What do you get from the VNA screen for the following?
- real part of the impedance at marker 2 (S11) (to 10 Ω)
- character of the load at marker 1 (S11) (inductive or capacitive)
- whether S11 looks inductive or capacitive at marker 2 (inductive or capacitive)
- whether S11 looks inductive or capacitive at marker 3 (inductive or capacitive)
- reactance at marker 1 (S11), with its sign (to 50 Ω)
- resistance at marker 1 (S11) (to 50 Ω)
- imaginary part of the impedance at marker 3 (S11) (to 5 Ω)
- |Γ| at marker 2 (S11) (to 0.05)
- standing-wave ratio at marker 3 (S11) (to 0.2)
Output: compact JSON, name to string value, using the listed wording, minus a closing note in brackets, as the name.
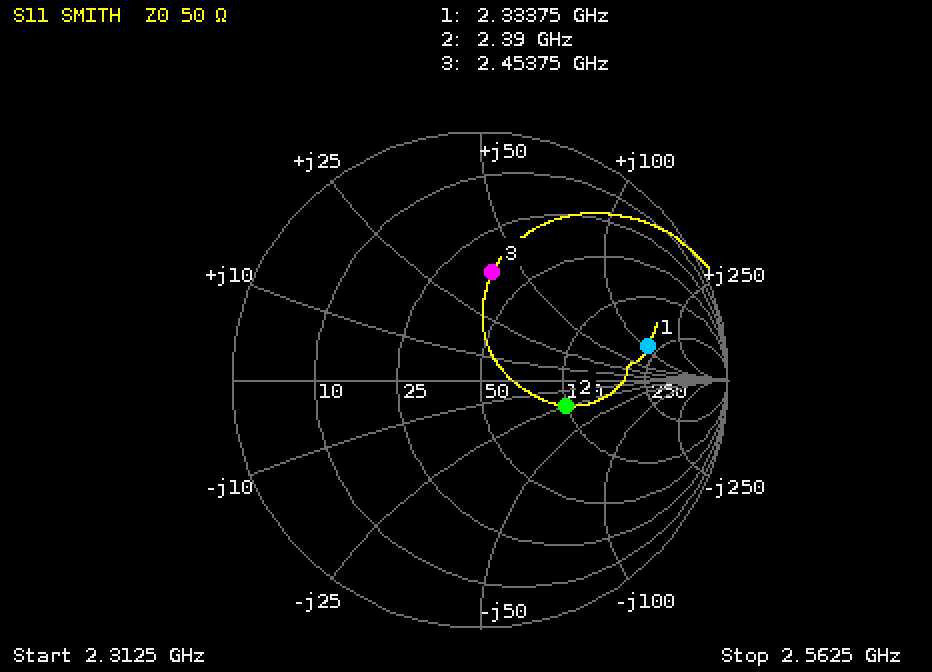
{"real part of the impedance at marker 2 (S11)": "100 Ω", "character of the load at marker 1 (S11)": "inductive", "whether S11 looks inductive or capacitive at marker 2": "capacitive", "whether S11 looks inductive or capacitive at marker 3": "inductive", "reactance at marker 1 (S11), with its sign": "+100 Ω", "resistance at marker 1 (S11)": "200 Ω", "imaginary part of the impedance at marker 3 (S11)": "+40 Ω", "|Γ| at marker 2 (S11)": "0.35", "standing-wave ratio at marker 3 (S11)": "2.6"}
